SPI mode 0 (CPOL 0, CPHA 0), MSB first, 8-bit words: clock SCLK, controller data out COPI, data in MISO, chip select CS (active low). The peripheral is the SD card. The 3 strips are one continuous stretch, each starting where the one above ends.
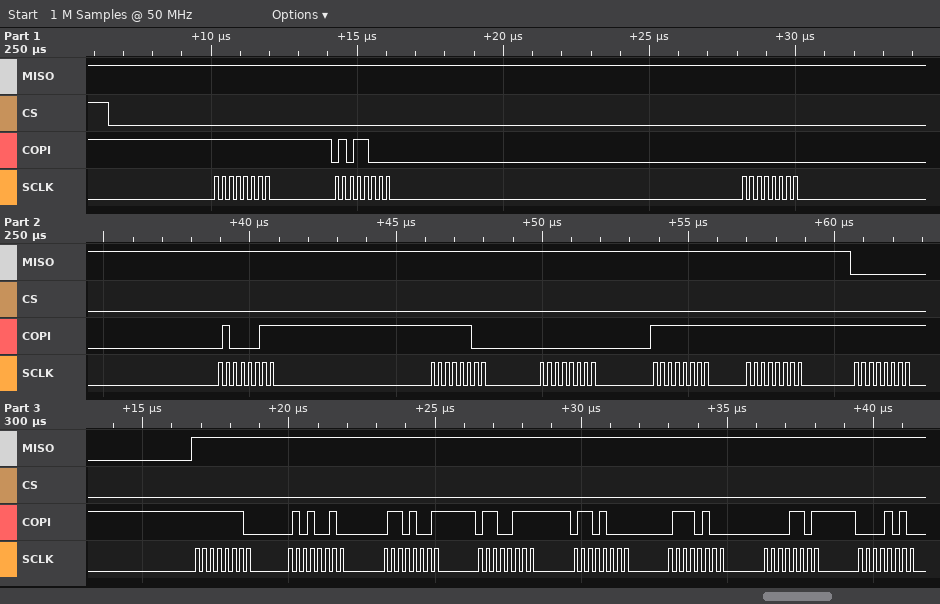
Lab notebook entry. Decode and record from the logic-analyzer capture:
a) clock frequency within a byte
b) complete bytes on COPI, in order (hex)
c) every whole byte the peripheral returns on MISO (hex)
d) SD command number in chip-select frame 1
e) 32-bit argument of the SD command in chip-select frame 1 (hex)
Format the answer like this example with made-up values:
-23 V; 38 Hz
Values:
4 MHz; FF 58 00 43 FC 00 FF FF FF FE 52 69 67 68 74 0D 0A; FF FF FF FF FF FF FF FF 00 FF FF FF FF FF FF FF FF; CMD24; 0x0043FC00
